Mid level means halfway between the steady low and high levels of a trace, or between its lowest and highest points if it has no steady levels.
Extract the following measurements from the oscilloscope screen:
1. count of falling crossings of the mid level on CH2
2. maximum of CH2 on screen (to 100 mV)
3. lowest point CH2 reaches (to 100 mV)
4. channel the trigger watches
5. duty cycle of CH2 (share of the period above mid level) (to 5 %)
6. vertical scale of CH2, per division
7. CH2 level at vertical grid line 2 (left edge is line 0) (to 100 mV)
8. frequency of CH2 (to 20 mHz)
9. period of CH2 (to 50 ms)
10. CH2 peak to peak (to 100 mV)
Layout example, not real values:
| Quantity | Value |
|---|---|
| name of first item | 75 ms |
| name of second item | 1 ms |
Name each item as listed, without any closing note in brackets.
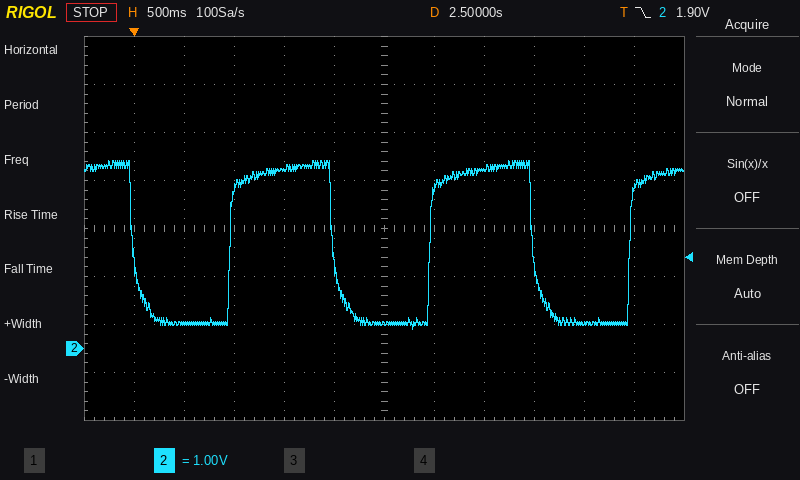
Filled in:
| Quantity | Value |
|---|---|
| count of falling crossings of the mid level on CH2 | 3 |
| maximum of CH2 on screen | 3.9 V |
| lowest point CH2 reaches | 400 mV |
| channel the trigger watches | CH2 |
| duty cycle of CH2 (share of the period above mid level) | 50 % |
| vertical scale of CH2, per division | 1 V |
| CH2 level at vertical grid line 2 (left edge is line 0) | 500 mV |
| frequency of CH2 | 500 mHz |
| period of CH2 | 2.00 s |
| CH2 peak to peak | 3.5 V |
